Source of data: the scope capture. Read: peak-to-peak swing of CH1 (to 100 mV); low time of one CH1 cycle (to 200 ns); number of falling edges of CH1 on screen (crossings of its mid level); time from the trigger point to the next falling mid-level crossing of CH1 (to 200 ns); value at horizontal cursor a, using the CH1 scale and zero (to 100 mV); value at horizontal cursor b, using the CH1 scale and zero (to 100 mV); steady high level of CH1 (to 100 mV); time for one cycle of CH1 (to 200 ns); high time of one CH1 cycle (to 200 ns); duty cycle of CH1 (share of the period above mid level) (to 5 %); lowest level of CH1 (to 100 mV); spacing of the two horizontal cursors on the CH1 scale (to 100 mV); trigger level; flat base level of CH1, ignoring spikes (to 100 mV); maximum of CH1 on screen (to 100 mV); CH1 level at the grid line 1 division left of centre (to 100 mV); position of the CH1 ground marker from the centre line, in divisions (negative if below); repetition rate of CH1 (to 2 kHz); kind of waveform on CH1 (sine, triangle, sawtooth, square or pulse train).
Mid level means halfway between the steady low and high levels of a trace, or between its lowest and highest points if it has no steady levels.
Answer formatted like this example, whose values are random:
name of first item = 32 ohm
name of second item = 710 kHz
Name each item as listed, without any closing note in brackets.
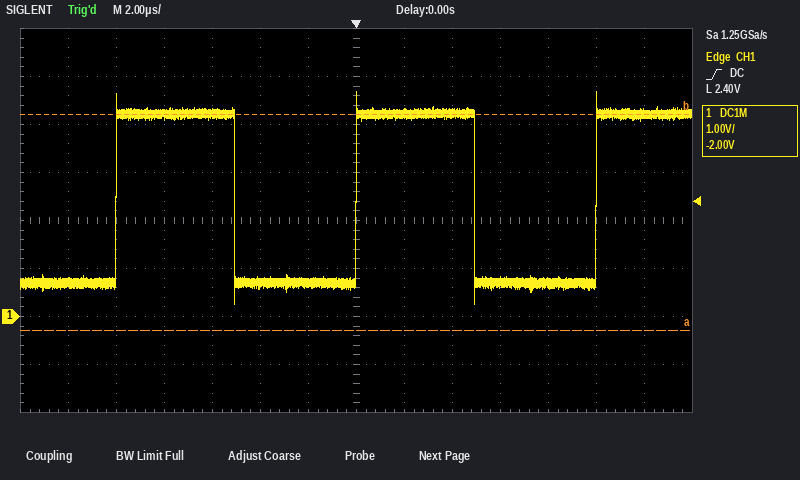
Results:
peak-to-peak swing of CH1 = 4.4 V
low time of one CH1 cycle = 5.0 µs
number of falling edges of CH1 on screen = 2
time from the trigger point to the next falling mid-level crossing of CH1 = 5.0 µs
value at horizontal cursor a, using the CH1 scale and zero = -300 mV
value at horizontal cursor b, using the CH1 scale and zero = 4.2 V
steady high level of CH1 = 4.2 V
time for one cycle of CH1 = 10.0 µs
high time of one CH1 cycle = 5.0 µs
duty cycle of CH1 (share of the period above mid level) = 50 %
lowest level of CH1 = 300 mV
spacing of the two horizontal cursors on the CH1 scale = 4.5 V
trigger level = 2.40 V
flat base level of CH1, ignoring spikes = 700 mV
maximum of CH1 on screen = 4.7 V
CH1 level at the grid line 1 division left of centre = 700 mV
position of the CH1 ground marker from the centre line, in divisions = -2.0 div
repetition rate of CH1 = 100 kHz
kind of waveform on CH1 = square
